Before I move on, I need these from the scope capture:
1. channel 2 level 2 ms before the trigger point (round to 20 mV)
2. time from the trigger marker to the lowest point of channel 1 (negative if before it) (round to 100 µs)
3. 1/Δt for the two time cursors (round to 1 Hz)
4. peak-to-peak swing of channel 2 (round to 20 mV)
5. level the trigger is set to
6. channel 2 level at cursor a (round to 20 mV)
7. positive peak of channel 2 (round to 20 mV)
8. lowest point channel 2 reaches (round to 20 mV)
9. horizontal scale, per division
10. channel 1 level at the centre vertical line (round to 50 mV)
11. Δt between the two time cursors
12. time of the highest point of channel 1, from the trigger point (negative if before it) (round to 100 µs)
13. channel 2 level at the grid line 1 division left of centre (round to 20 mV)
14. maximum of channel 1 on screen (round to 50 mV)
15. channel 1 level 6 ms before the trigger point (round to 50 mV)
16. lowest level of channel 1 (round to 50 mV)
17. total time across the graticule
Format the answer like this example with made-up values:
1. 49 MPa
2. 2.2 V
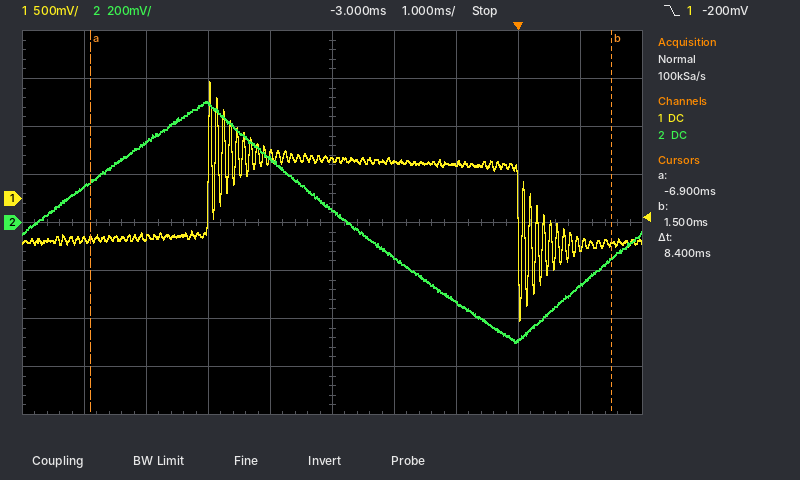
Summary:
1. -140 mV
2. 0.0 ms
3. 119 Hz
4. 1.00 V
5. -200 mV
6. 160 mV
7. 500 mV
8. -500 mV
9. 1 ms
10. 400 mV
11. 8.4 ms
12. -5.0 ms
13. 260 mV
14. 1.20 V
15. -400 mV
16. -1.25 V
17. 10 ms
